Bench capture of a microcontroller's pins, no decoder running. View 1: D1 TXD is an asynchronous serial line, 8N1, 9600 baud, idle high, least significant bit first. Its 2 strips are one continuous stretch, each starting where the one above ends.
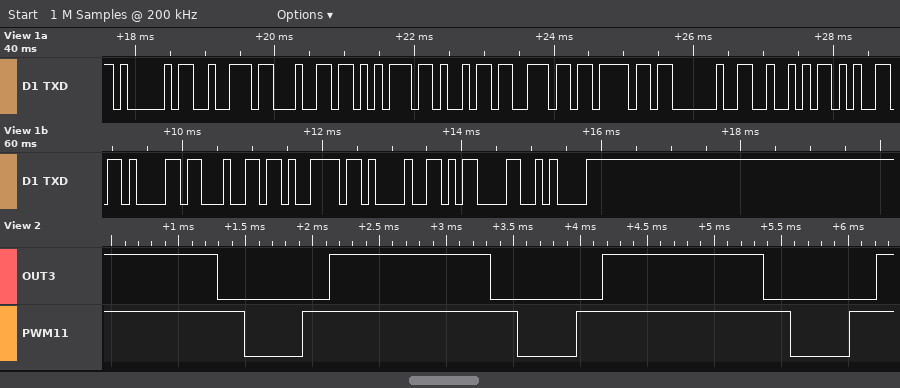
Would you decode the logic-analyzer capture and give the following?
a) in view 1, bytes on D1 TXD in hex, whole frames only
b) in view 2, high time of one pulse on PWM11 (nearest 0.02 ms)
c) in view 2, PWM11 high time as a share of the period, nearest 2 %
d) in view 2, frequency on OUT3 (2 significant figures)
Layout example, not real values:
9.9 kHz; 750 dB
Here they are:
41 72 64 75 69 6E 6F 20 52 65 61 64 79 21 0D 0A; 1.60 ms; 78 %; 490 Hz
